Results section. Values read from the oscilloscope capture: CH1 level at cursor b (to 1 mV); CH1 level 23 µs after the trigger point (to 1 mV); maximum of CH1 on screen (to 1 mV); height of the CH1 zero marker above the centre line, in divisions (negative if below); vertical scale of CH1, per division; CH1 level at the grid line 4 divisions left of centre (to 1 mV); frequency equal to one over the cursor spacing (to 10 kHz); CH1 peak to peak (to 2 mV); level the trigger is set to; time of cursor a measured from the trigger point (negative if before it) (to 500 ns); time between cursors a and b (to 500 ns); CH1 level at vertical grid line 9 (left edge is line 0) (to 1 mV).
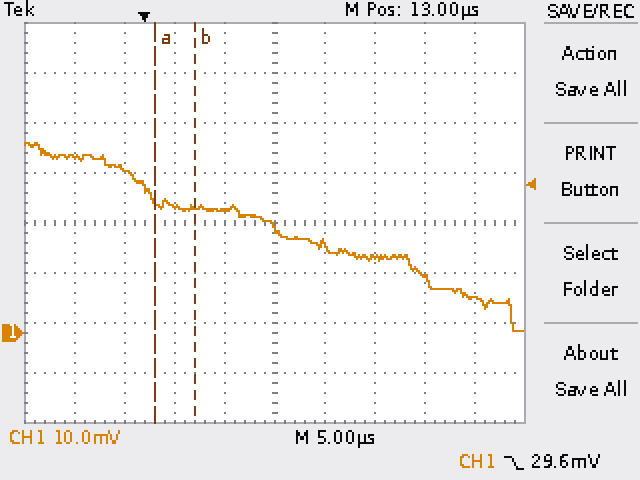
25 mV
15 mV
38 mV
-2.2 div
10 mV
35 mV
250 kHz
38 mV
29.6 mV
+1.0 µs
4.0 µs
7 mV
